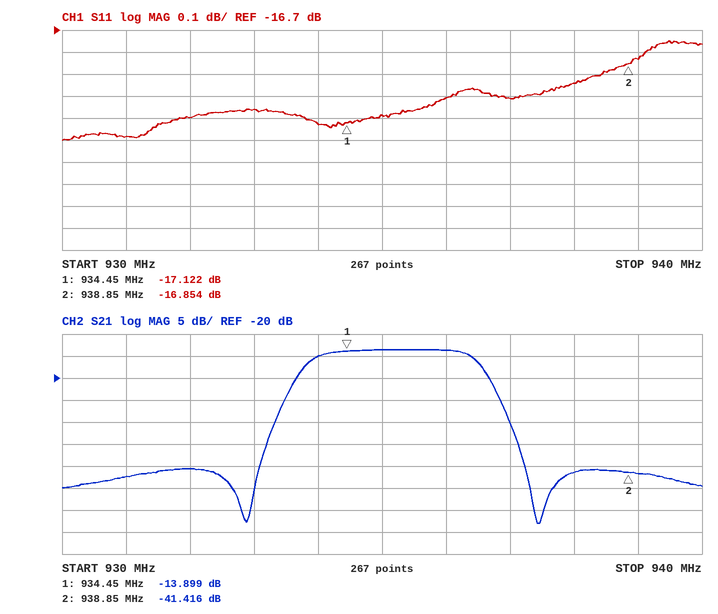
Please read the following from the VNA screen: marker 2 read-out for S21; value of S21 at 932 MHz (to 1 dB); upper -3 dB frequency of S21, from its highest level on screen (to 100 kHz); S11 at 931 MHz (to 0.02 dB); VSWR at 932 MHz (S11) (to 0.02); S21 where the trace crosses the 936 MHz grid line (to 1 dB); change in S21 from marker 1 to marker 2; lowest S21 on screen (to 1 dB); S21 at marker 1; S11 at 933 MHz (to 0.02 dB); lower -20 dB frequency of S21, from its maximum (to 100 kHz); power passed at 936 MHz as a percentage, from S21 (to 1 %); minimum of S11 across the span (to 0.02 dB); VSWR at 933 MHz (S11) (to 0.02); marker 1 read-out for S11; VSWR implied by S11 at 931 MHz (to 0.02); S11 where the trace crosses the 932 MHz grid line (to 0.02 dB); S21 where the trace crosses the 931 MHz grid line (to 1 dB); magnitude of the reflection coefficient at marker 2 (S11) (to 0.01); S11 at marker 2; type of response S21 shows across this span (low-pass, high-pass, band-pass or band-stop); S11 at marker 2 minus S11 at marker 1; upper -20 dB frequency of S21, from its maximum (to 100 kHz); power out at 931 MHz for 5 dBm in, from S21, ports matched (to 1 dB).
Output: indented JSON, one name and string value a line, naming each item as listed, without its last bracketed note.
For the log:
{
  "marker 2 read-out for S21": "-41.416 dB",
  "value of S21 at 932 MHz": "-41 dB",
  "upper -3 dB frequency of S21, from its highest level on screen": "936.5 MHz",
  "S11 at 931 MHz": "-17.18 dB",
  "VSWR at 932 MHz (S11)": "1.32",
  "S21 where the trace crosses the 936 MHz grid line": "-14 dB",
  "change in S21 from marker 1 to marker 2": "-27.517 dB",
  "lowest S21 on screen": "-53 dB",
  "S21 at marker 1": "-13.899 dB",
  "S11 at 933 MHz": "-17.06 dB",
  "lower -20 dB frequency of S21, from its maximum": "933.2 MHz",
  "power passed at 936 MHz as a percentage, from S21": "4 %",
  "minimum of S11 across the span": "-17.20 dB",
  "VSWR at 933 MHz (S11)": "1.32",
  "marker 1 read-out for S11": "-17.122 dB",
  "VSWR implied by S11 at 931 MHz": "1.32",
  "S11 where the trace crosses the 932 MHz grid line": "-17.10 dB",
  "S21 where the trace crosses the 931 MHz grid line": "-42 dB",
  "magnitude of the reflection coefficient at marker 2 (S11)": "0.14",
  "S11 at marker 2": "-16.854 dB",
  "type of response S21 shows across this span": "band-pass",
  "S11 at marker 2 minus S11 at marker 1": "0.268 dB",
  "upper -20 dB frequency of S21, from its maximum": "937.1 MHz",
  "power out at 931 MHz for 5 dBm in, from S21, ports matched": "-37 dBm"
}
